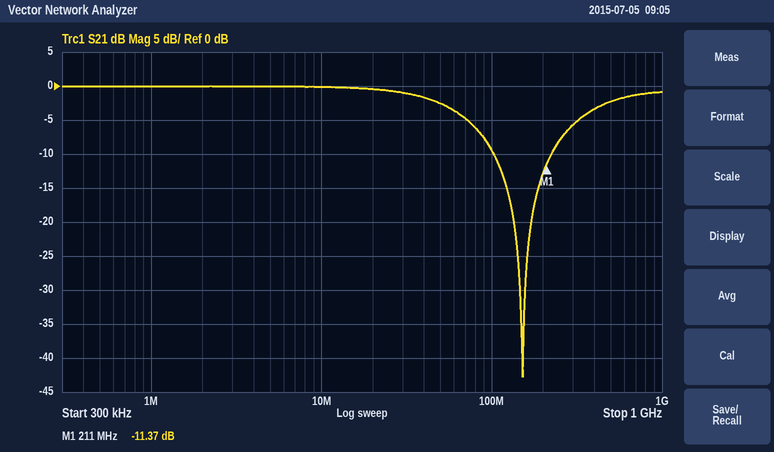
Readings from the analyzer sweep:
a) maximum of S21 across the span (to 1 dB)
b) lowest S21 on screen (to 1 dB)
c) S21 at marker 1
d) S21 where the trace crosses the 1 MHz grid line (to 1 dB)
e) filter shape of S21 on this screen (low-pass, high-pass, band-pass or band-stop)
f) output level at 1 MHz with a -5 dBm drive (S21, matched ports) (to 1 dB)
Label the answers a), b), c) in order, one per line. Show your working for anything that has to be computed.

a) 0 dB
b) -43 dB
c) -11.37 dB
d) 0 dB
e) band-stop
f) -5 dBm + (0 dB) = -5 dBm
